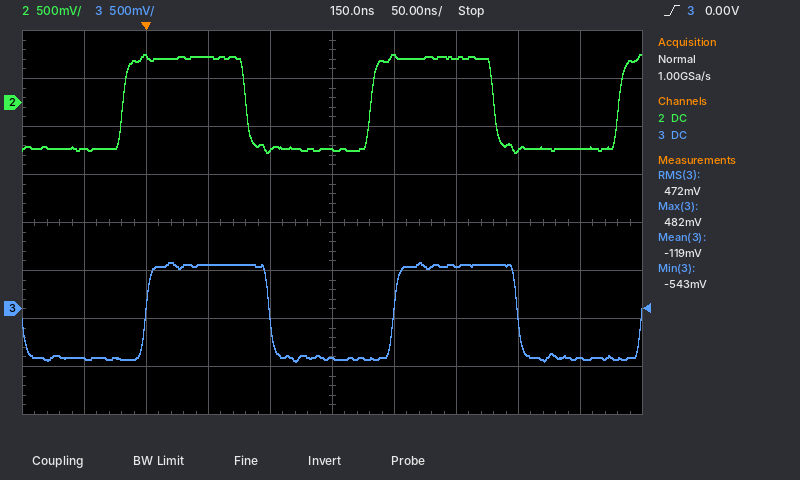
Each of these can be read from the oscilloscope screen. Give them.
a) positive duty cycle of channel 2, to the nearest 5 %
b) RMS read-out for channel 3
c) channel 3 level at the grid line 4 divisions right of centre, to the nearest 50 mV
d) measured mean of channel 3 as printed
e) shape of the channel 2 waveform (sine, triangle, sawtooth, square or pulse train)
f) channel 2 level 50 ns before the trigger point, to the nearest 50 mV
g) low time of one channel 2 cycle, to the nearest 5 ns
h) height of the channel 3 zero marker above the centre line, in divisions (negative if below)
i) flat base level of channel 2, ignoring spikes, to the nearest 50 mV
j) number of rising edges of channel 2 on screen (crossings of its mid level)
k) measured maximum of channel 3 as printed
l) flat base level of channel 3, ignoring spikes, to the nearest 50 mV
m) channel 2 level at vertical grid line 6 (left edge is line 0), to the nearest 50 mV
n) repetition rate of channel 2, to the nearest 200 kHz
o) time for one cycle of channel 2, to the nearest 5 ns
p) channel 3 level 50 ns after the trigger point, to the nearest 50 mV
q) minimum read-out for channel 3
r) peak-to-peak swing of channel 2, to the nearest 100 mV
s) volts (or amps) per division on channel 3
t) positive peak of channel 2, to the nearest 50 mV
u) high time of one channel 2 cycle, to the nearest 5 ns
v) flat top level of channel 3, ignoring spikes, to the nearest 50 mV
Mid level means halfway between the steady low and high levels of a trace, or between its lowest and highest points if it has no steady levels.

50 %
472 mV
-500 mV
-119 mV
square
-500 mV
100 ns
-1.8 div
-500 mV
3
482 mV
-500 mV
500 mV
5.0 MHz
200 ns
450 mV
-543 mV
1.00 V
500 mV
500 mV
100 ns
450 mV
